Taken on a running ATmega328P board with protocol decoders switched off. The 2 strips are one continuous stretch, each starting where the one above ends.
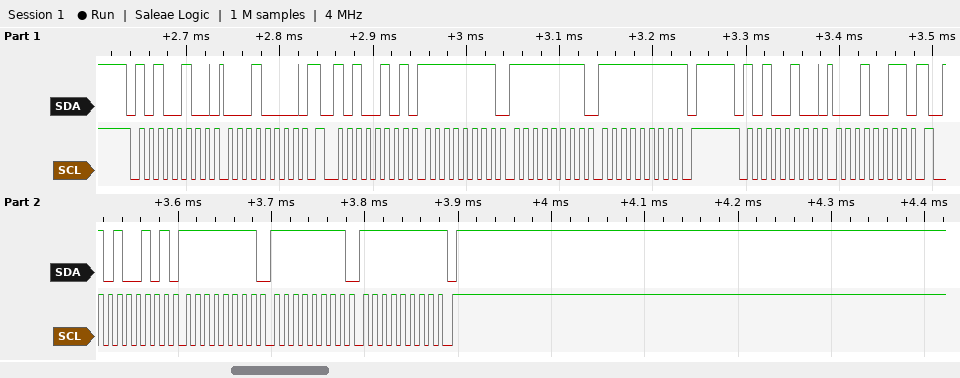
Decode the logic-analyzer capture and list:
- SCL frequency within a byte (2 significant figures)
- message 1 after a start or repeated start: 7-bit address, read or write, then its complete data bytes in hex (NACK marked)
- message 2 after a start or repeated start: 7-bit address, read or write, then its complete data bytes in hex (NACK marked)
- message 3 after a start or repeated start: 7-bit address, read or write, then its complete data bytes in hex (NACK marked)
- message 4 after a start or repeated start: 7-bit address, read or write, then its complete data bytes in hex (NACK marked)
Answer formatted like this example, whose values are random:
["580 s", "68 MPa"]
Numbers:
["100 kHz", "0x52 write: 10", "0x52 read: FF FF FF NACK", "0x52 write: 13", "0x52 read: FF FF FF NACK"]
